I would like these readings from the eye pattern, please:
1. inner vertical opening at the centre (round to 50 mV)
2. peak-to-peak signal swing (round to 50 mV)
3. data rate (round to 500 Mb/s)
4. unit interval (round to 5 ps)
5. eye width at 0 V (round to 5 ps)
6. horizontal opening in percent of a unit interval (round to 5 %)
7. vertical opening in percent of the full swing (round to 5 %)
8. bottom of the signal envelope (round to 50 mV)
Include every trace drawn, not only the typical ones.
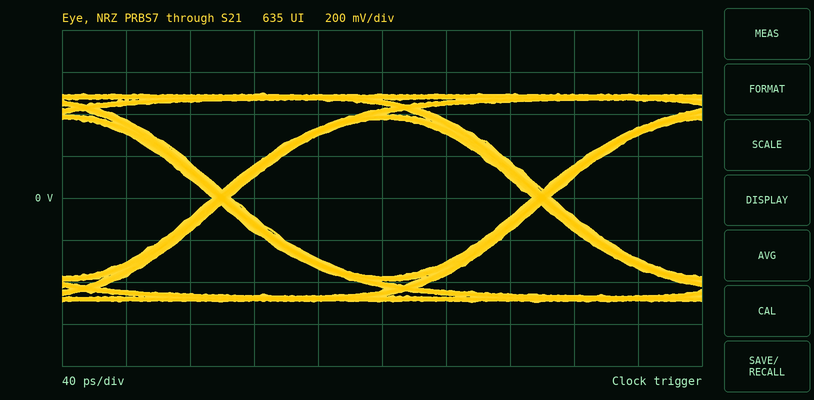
750 mV
1.00 V
5.0 Gb/s
200 ps
190 ps
95 %
75 %
-500 mV
